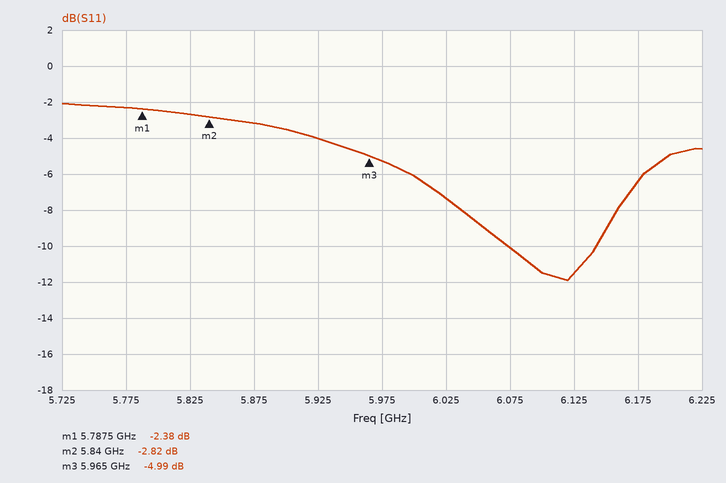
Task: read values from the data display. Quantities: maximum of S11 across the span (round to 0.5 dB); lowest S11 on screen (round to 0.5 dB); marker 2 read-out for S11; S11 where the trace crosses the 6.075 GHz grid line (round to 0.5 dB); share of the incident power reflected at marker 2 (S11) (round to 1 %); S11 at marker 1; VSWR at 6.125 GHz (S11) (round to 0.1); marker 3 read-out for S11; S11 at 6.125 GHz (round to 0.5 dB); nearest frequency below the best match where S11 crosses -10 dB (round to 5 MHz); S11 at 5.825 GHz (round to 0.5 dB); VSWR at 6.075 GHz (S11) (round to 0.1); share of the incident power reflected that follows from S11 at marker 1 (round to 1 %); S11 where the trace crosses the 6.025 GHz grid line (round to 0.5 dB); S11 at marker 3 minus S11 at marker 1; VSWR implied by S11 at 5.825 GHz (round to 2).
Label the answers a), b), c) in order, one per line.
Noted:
a) -2.0 dB
b) -12.0 dB
c) -2.82 dB
d) -10.0 dB
e) 52 %
f) -2.38 dB
g) 1.7
h) -4.99 dB
i) -11.5 dB
j) 6.075 GHz
k) -2.5 dB
l) 1.9
m) 58 %
n) -7.5 dB
o) -2.61 dB
p) 6
